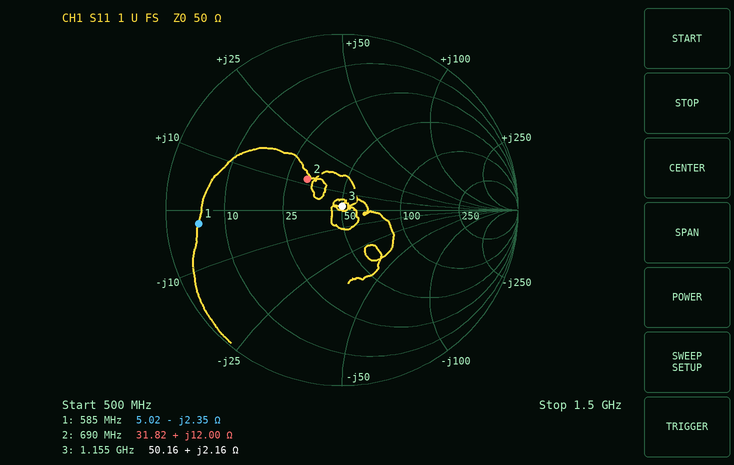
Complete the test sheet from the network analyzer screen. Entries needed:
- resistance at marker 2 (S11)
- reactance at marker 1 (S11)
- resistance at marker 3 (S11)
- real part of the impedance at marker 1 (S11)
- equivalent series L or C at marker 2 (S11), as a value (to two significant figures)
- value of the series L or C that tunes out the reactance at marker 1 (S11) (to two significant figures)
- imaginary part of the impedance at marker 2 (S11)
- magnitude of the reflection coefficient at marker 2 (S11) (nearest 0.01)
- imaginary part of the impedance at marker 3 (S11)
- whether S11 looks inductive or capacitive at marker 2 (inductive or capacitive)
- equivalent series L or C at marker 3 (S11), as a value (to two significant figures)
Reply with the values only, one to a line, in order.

31.82 Ω
-2.35 Ω
50.16 Ω
5.02 Ω
2.8 nH
640 pH
+12.00 Ω
0.26
+2.16 Ω
inductive
300 pH
